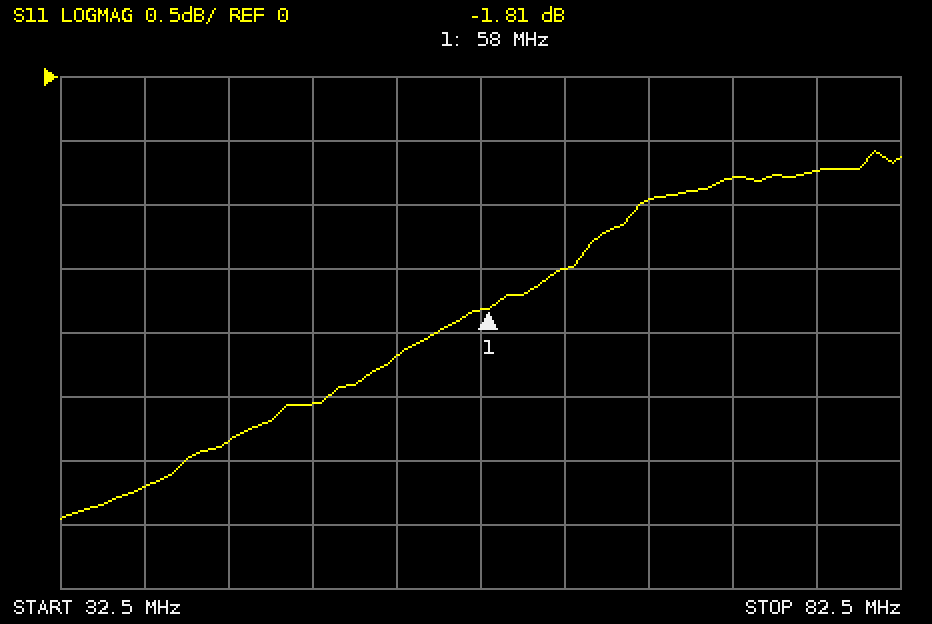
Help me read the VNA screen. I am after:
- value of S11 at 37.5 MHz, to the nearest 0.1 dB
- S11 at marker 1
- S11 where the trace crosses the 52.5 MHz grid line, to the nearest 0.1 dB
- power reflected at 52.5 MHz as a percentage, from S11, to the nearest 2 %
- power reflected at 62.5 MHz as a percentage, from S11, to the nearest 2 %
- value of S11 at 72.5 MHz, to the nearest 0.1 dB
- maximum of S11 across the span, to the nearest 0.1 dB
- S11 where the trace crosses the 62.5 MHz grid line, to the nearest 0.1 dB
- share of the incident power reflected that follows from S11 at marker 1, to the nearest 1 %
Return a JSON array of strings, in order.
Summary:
["-3.2 dB", "-1.81 dB", "-2.2 dB", "60 %", "70 %", "-0.8 dB", "-0.6 dB", "-1.5 dB", "66 %"]
